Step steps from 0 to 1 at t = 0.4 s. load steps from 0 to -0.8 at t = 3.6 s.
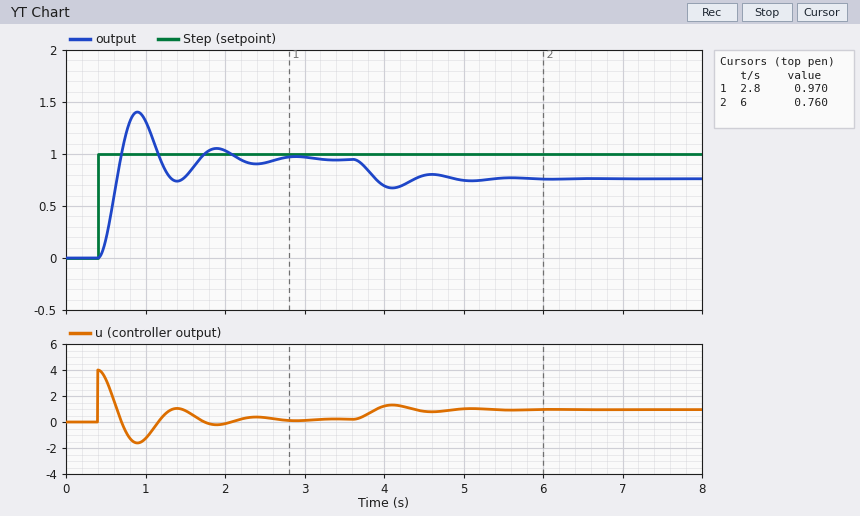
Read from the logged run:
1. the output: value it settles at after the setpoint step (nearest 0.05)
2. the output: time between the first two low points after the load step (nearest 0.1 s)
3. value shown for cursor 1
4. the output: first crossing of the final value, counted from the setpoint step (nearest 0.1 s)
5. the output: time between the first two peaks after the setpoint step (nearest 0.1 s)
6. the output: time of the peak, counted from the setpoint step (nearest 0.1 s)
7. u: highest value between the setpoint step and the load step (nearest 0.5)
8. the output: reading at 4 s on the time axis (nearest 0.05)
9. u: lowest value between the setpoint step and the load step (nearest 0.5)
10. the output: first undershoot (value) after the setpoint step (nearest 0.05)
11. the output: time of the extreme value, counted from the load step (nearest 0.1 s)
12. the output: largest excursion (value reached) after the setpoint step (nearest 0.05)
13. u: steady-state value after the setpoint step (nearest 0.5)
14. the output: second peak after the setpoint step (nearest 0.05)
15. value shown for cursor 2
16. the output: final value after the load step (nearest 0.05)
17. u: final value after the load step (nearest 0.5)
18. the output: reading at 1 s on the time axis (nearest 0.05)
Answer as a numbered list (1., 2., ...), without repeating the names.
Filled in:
1. 0.95
2. 1.0 s
3. 0.970
4. 0.3 s
5. 1.0 s
6. 0.5 s
7. 4.0
8. 0.70
9. -1.5
10. 0.75
11. 0.5 s
12. 1.40
13. 0.0
14. 1.05
15. 0.760
16. 0.75
17. 1.0
18. 1.30
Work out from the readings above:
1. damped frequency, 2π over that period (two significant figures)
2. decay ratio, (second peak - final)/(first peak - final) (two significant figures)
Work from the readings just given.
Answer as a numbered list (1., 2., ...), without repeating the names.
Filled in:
1. 6.3 rad/s
2. 0.22
